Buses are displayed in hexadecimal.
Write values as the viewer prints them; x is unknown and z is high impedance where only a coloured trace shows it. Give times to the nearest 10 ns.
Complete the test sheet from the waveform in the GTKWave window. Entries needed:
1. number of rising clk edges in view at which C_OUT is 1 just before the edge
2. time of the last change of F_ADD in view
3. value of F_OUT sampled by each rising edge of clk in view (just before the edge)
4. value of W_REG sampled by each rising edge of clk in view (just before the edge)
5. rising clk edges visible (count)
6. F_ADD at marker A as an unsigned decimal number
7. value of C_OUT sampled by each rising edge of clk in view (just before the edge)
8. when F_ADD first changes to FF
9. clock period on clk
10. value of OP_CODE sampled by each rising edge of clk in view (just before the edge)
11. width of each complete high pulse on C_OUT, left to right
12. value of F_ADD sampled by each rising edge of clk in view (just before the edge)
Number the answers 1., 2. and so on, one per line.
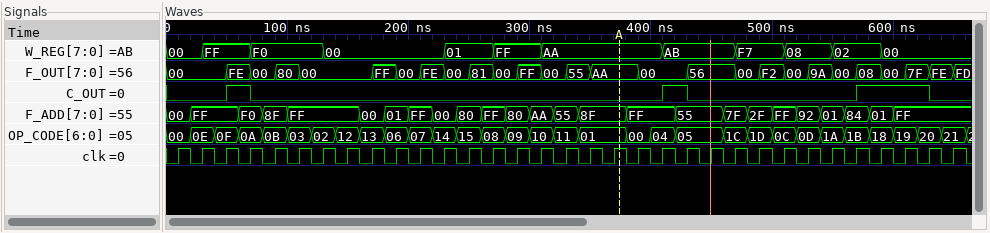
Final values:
1. 5
2. 600 ns
3. 00, 00, 00, FE, 00, 80, 00, 00, 00, FF, 00, FE, 00, 81, 00, FF, 00, 55, AA, AA, 00, 00, 56, 56, 00, F2, 00, 9A, 00, 08, 00, 7F, FE
4. 00, 00, FF, FF, F0, F0, F0, 00, 00, 00, 00, 00, 01, 01, FF, FF, AA, AA, AA, AA, AA, AB, AB, AB, F7, F7, 08, 08, 02, 02, 00, 00, 00
5. 33
6. 143
7. 0 0 0 1 0 0 0 0 0 0 0 0 0 0 0 0 0 0 0 0 0 1 0 0 0 0 0 0 0 1 1 1 0
8. 20 ns
9. 20 ns
10. 00, 0E, 0F, 0A, 0B, 03, 02, 12, 13, 06, 07, 14, 15, 08, 09, 10, 11, 01, 01, 00, 04, 05, 05, 1C, 1D, 0C, 0D, 1A, 1B, 18, 19, 20, 21
11. 20 ns, 20 ns, 60 ns
12. 00, FF, FF, F0, 8F, FF, FF, FF, 00, 01, FF, 00, 80, FF, 80, AA, 55, 8F, 8F, FF, FF, 55, 55, 7F, 2F, FF, 92, 01, 84, 01, FF, FF, FF
